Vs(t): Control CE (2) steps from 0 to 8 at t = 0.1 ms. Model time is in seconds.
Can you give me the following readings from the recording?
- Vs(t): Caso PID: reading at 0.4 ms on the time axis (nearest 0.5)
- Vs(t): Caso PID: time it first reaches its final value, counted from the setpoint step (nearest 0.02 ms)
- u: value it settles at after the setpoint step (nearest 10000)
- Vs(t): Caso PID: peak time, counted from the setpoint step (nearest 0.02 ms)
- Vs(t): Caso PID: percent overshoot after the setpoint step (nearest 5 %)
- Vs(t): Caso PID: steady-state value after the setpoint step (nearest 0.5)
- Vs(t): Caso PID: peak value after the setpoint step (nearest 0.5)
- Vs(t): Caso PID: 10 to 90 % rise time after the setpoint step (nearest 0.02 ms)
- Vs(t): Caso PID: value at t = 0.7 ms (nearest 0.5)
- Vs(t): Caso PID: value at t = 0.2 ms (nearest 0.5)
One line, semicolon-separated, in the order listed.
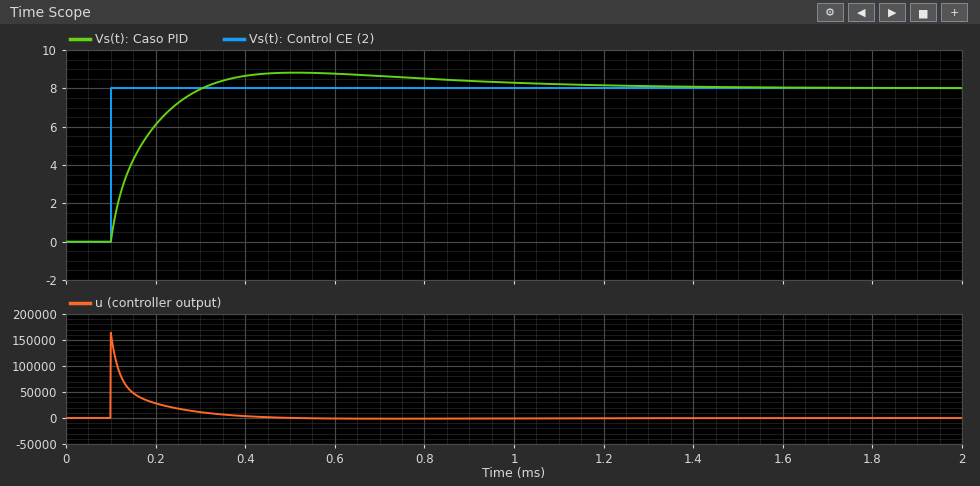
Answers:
8.5; 0.20 ms; 0; 0.42 ms; 10 %; 8.0; 9.0; 0.14 ms; 8.5; 6.0
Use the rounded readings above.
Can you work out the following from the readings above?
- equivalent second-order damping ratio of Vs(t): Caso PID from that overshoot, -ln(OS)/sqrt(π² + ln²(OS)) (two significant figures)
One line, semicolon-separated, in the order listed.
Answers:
0.59
